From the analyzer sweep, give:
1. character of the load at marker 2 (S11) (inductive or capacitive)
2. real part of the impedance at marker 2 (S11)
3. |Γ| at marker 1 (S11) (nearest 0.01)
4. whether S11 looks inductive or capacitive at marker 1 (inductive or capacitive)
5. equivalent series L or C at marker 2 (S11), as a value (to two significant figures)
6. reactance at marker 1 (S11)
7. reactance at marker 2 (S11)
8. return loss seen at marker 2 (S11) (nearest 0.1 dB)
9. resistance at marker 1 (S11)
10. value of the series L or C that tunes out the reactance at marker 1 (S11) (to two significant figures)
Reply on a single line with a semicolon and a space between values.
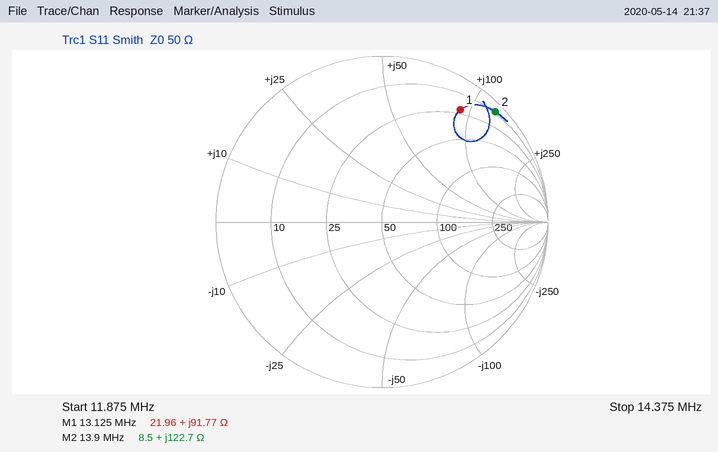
inductive; 8.5 Ω; 0.82; inductive; 1.4 µH; +91.77 Ω; +122.7 Ω; 0.4 dB; 21.96 Ω; 130 pF
